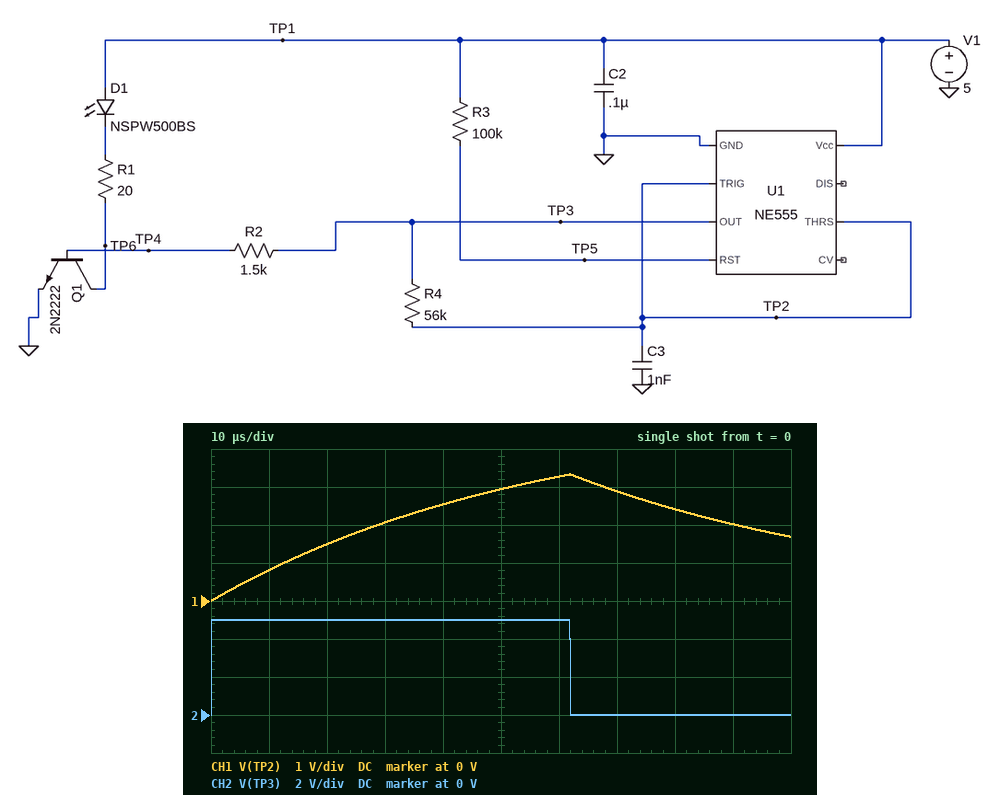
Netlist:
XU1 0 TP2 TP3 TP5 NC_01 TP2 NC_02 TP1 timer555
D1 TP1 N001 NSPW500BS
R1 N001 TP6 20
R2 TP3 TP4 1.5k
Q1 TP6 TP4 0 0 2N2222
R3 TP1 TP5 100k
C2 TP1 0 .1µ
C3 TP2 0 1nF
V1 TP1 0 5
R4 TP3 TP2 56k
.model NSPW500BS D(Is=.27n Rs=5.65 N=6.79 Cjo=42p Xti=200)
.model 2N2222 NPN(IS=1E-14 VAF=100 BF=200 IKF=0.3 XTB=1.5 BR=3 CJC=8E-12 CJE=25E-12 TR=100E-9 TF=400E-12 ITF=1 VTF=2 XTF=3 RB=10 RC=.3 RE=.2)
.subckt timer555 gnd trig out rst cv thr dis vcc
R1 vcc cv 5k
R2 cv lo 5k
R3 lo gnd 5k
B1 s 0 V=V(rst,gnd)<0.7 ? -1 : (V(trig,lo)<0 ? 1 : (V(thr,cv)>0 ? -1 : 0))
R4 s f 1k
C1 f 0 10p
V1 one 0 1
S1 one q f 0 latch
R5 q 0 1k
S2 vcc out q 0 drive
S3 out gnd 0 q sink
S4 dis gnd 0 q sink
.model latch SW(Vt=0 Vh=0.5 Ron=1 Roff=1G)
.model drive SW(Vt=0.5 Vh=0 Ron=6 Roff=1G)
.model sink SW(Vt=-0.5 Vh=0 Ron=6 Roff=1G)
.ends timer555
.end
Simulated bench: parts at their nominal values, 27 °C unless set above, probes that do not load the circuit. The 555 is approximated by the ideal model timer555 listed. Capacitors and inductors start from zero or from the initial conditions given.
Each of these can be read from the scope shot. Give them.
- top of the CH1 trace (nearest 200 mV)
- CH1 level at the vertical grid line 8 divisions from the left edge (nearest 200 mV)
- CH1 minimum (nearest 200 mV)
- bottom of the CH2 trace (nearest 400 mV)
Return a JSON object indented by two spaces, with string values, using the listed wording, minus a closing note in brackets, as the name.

{
  "top of the CH1 trace": "3.4 V",
  "CH1 level at the vertical grid line 8 divisions from the left edge": "2.4 V",
  "CH1 minimum": "0 V",
  "bottom of the CH2 trace": "0 V"
}
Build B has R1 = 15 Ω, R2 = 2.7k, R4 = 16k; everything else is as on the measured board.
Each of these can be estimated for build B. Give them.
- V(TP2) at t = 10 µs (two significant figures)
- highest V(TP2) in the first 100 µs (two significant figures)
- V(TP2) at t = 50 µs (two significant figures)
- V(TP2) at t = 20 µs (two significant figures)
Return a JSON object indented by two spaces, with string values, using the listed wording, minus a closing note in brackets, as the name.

{
  "V(TP2) at t = 10 µs": "2.3 V",
  "highest V(TP2) in the first 100 µs": "3.3 V",
  "V(TP2) at t = 50 µs": "1.8 V",
  "V(TP2) at t = 20 µs": "2.9 V"
}
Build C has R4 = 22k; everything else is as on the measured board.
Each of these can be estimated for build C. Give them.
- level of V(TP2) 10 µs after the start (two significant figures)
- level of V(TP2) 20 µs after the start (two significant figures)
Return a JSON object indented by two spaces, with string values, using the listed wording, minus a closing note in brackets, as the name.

{
  "level of V(TP2) 10 µs after the start": "1.8 V",
  "level of V(TP2) 20 µs after the start": "3.0 V"
}
